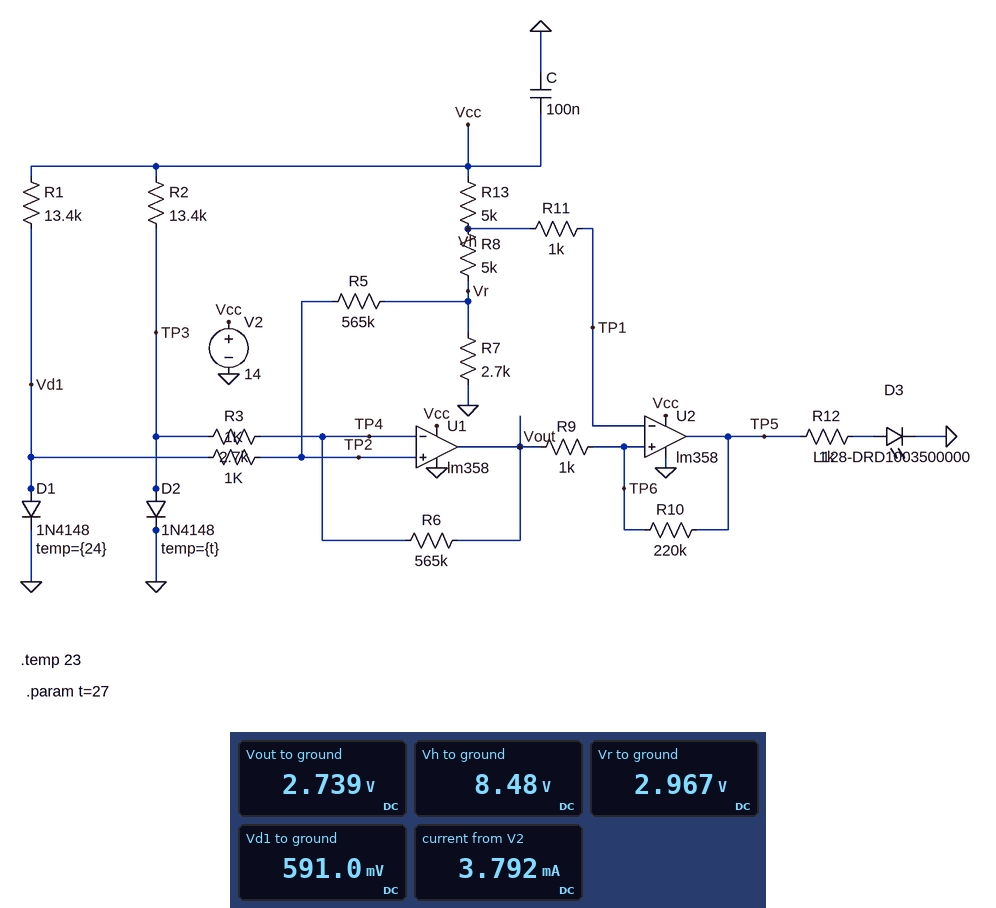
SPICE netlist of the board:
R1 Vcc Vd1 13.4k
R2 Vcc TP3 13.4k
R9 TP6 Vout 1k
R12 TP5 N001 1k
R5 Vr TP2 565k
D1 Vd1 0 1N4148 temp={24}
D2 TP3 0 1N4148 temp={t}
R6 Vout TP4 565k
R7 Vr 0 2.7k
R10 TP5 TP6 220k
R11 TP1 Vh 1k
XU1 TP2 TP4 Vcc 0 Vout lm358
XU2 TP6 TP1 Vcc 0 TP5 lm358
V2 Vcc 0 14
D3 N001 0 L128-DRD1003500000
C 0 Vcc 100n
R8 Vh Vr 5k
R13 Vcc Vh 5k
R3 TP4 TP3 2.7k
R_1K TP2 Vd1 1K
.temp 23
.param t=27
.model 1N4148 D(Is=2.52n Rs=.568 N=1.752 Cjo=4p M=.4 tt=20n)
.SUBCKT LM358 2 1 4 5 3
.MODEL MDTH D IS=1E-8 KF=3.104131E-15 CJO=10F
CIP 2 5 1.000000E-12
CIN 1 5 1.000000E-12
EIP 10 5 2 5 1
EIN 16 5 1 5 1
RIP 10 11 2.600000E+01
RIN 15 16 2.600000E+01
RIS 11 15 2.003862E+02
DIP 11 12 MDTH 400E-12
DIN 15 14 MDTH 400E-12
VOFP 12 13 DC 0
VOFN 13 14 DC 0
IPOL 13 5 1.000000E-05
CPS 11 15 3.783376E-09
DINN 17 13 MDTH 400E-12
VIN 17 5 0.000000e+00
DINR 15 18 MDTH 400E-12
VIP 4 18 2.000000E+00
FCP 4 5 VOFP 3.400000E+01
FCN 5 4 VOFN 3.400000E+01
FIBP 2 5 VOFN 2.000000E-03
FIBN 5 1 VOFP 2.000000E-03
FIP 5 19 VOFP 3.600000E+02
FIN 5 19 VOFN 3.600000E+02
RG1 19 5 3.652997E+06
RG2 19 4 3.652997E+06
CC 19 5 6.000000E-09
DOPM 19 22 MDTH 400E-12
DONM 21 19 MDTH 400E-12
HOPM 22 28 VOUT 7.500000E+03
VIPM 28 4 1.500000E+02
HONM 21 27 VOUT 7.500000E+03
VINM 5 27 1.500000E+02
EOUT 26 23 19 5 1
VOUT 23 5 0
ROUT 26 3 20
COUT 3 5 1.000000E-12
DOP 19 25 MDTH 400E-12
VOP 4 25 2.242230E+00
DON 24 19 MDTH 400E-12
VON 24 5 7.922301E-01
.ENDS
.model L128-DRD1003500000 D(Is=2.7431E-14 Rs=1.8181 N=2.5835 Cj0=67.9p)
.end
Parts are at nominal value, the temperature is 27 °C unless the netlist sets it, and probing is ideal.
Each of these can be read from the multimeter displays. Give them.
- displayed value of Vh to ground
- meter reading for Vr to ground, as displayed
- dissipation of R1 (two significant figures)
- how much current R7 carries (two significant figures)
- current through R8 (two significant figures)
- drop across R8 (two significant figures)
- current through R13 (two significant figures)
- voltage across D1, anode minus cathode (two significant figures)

8.48 V
2.967 V
13 mW
1.1 mA
1.1 mA
5.5 V
1.1 mA
590 mV
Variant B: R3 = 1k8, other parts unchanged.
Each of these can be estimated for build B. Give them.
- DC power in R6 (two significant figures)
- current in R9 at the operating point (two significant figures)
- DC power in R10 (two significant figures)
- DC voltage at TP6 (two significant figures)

18 µW
18 µA
68 µW
3.8 V
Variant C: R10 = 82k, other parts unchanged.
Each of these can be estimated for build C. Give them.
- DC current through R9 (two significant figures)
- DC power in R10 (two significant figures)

34 µA
96 µW
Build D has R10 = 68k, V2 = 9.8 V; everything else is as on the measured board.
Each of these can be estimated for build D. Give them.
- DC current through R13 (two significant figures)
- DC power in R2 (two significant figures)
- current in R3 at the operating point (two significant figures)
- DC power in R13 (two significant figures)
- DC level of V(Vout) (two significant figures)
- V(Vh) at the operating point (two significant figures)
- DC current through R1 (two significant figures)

770 µA
6.4 mW
3.3 µA
3.0 mW
2.4 V
5.9 V
690 µA
